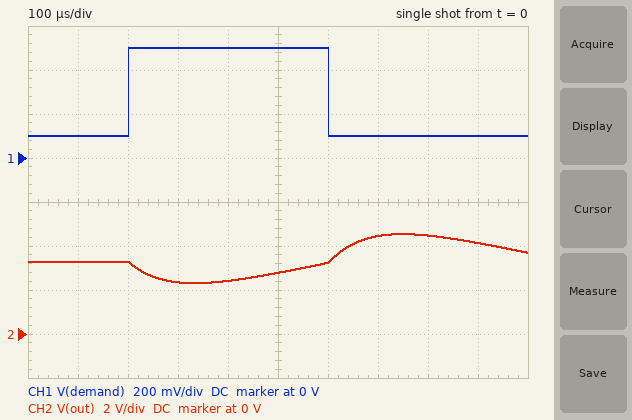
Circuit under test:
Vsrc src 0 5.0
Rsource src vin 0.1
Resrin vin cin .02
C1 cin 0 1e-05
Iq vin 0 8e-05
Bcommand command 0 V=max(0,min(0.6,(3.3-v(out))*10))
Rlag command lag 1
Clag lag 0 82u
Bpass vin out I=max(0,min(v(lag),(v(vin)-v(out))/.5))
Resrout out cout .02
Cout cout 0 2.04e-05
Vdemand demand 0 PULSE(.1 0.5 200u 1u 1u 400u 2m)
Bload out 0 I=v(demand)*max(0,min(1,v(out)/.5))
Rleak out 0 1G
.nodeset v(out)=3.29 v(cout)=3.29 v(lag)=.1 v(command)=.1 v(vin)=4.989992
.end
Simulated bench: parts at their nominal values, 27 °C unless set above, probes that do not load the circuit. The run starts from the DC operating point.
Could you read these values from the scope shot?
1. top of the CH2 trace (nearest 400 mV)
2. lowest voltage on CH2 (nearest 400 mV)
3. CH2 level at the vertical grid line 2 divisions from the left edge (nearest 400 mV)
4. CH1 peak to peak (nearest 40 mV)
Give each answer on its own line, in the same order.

4.4 V
2.4 V
3.2 V
400 mV
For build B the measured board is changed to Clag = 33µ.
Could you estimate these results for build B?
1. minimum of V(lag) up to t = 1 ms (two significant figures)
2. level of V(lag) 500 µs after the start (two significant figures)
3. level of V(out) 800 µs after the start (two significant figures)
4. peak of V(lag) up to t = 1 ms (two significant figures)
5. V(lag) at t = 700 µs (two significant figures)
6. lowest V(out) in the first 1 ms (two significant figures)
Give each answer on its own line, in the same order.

4.4 mV
490 mV
3.3 V
600 mV
26 mV
2.9 V
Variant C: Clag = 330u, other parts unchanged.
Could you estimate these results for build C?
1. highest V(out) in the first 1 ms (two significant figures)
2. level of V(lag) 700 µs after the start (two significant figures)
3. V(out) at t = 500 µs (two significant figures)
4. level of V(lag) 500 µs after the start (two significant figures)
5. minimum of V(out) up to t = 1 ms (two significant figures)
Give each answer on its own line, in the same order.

4.9 V
490 mV
390 mV
400 mV
370 mV
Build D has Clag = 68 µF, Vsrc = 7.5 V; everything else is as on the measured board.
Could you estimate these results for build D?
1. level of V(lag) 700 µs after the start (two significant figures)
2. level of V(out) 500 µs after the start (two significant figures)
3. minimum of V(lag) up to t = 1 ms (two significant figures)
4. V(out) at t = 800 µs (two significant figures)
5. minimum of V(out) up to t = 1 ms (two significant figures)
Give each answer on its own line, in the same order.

120 mV
3.1 V
4.1 mV
3.9 V
2.5 V
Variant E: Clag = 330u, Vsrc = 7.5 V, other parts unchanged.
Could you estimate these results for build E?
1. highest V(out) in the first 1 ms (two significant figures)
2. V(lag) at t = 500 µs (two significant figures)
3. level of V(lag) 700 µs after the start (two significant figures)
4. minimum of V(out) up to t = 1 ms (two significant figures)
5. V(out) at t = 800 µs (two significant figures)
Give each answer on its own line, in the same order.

6.4 V
400 mV
490 mV
370 mV
4.1 V
